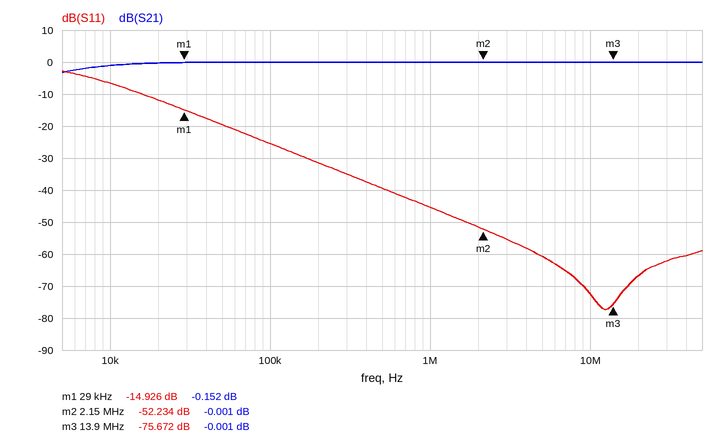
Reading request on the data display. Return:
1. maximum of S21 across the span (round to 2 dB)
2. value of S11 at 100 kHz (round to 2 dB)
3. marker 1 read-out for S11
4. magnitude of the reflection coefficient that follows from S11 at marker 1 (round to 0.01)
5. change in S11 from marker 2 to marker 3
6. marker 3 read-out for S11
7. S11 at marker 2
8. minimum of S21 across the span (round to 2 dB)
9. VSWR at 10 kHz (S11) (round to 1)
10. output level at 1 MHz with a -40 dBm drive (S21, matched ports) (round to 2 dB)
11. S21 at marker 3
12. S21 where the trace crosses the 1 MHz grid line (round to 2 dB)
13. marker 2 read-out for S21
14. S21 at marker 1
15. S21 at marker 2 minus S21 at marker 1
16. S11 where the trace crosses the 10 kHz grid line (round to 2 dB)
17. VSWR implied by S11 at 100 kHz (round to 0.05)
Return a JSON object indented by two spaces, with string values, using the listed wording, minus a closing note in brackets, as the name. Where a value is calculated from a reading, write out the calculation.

{
  "maximum of S21 across the span": "0 dB",
  "value of S11 at 100 kHz": "-26 dB",
  "marker 1 read-out for S11": "-14.926 dB",
  "magnitude of the reflection coefficient that follows from S11 at marker 1": "10^(-14.926/20) ≈ 0.18",
  "change in S11 from marker 2 to marker 3": "-75.672 − (-52.234) = -23.438 dB",
  "marker 3 read-out for S11": "-75.672 dB",
  "S11 at marker 2": "-52.234 dB",
  "minimum of S21 across the span": "-4 dB",
  "VSWR at 10 kHz (S11)": "|Γ| = 10^(-6/20) = 0.5012; VSWR = (1 + 0.5012)/(1 − 0.5012) ≈ 3",
  "output level at 1 MHz with a -40 dBm drive (S21, matched ports)": "-40 dBm + (0 dB) = -40 dBm",
  "S21 at marker 3": "-0.001 dB",
  "S21 where the trace crosses the 1 MHz grid line": "0 dB",
  "marker 2 read-out for S21": "-0.001 dB",
  "S21 at marker 1": "-0.152 dB",
  "S21 at marker 2 minus S21 at marker 1": "-0.001 − (-0.152) = 0.151 dB",
  "S11 where the trace crosses the 10 kHz grid line": "-6 dB",
  "VSWR implied by S11 at 100 kHz": "|Γ| = 10^(-26/20) = 0.0501; VSWR = (1 + 0.0501)/(1 − 0.0501) ≈ 1.11, so 1.10 to the nearest 0.05"
}
